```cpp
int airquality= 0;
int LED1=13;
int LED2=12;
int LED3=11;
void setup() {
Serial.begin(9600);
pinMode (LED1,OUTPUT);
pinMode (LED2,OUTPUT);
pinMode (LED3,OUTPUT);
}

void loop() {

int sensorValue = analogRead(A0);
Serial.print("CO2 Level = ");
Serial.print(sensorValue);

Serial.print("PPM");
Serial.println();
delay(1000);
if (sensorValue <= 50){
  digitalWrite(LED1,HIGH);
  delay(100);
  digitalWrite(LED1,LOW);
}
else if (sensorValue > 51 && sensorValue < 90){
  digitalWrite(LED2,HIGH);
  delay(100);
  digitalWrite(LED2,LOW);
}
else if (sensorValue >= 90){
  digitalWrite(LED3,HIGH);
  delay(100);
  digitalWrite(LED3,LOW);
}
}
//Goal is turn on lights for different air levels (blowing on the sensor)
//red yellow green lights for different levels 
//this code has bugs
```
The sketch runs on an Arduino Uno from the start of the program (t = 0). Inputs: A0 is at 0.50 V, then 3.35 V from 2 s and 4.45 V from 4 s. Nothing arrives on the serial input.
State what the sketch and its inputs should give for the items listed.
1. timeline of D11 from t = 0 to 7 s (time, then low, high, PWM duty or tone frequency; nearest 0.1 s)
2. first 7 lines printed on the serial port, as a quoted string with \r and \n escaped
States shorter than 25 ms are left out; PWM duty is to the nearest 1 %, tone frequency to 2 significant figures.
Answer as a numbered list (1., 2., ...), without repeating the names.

1. 0 s low; 1 s high; 1.1 s low; 2.1 s high; 2.2 s low; 3.2 s high; 3.3 s low; 4.3 s high; 4.4 s low; 5.4 s high; 5.5 s low; 6.5 s high; 6.6 s low
2. "CO2 Level = 102PPM\r\nCO2 Level = 102PPM\r\nCO2 Level = 686PPM\r\nCO2 Level = 686PPM\r\nCO2 Level = 911PPM\r\nCO2 Level = 911PPM\r\nCO2 Level = 911PPM\r\n"
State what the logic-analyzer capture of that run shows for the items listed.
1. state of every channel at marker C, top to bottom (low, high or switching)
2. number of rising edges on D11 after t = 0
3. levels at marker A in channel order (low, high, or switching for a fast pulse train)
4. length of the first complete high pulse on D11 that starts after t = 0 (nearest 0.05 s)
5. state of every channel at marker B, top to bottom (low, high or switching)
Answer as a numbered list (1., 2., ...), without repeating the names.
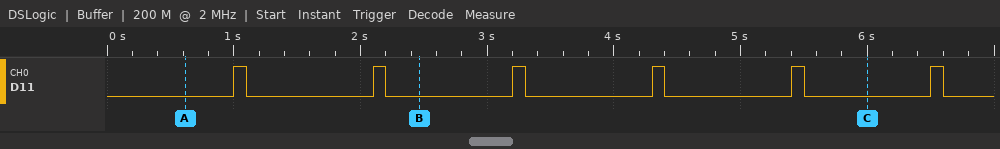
1. D11 low
2. 6
3. D11 low
4. 0.10 s
5. D11 low
